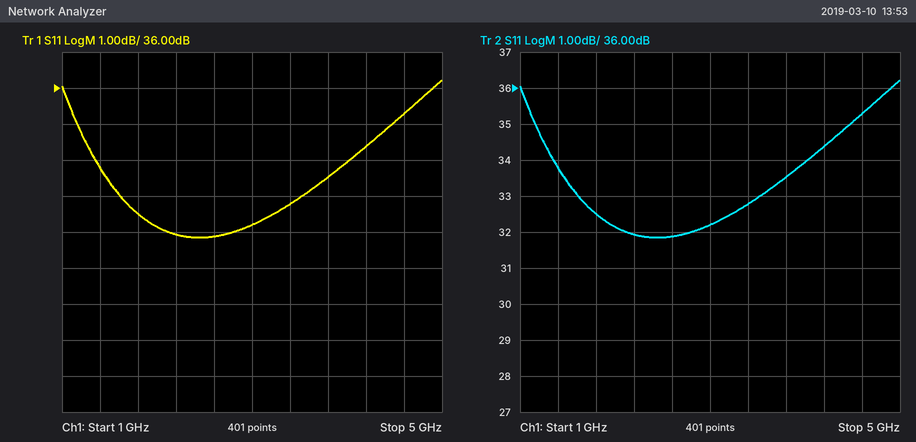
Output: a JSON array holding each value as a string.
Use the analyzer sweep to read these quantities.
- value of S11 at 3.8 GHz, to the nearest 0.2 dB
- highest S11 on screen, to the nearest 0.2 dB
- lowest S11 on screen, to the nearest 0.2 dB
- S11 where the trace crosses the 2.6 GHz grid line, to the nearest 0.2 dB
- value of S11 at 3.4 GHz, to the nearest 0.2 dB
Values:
["33.6 dB", "36.2 dB", "31.8 dB", "31.8 dB", "32.8 dB"]
